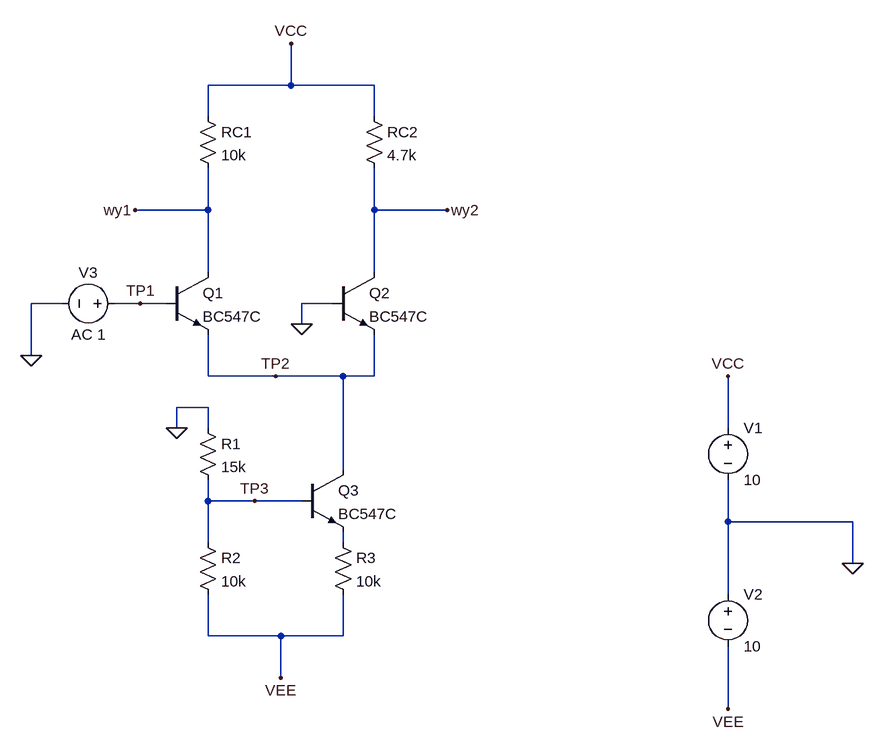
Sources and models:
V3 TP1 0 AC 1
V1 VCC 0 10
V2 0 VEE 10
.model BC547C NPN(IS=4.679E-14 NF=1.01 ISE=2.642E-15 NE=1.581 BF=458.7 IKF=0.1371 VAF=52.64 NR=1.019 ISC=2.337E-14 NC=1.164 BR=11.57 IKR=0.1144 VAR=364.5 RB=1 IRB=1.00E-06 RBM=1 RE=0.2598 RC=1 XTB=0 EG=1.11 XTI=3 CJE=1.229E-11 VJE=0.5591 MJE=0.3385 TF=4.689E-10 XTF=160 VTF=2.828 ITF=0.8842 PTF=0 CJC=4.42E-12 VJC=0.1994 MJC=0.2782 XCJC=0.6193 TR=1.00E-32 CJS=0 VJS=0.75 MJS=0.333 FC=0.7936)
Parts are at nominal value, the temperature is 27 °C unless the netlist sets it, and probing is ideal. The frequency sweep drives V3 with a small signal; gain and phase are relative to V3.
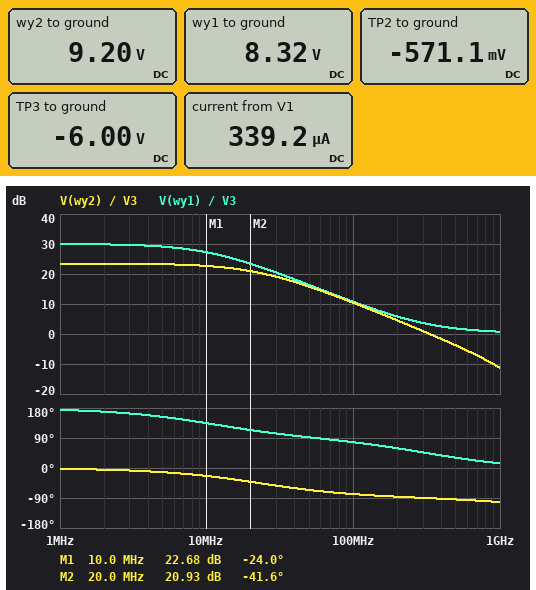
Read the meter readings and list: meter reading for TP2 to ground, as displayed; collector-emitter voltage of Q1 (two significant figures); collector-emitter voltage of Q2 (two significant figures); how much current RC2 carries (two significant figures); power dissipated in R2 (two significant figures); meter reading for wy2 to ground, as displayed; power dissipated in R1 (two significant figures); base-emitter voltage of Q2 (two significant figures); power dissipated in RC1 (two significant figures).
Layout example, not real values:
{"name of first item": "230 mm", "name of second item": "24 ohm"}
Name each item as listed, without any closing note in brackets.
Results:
{"meter reading for TP2 to ground, as displayed": "-571.1 mV", "collector-emitter voltage of Q1": "8.9 V", "collector-emitter voltage of Q2": "9.8 V", "how much current RC2 carries": "170 µA", "power dissipated in R2": "1.6 mW", "meter reading for wy2 to ground, as displayed": "9.20 V", "power dissipated in R1": "2.4 mW", "base-emitter voltage of Q2": "570 mV", "power dissipated in RC1": "280 µW"}
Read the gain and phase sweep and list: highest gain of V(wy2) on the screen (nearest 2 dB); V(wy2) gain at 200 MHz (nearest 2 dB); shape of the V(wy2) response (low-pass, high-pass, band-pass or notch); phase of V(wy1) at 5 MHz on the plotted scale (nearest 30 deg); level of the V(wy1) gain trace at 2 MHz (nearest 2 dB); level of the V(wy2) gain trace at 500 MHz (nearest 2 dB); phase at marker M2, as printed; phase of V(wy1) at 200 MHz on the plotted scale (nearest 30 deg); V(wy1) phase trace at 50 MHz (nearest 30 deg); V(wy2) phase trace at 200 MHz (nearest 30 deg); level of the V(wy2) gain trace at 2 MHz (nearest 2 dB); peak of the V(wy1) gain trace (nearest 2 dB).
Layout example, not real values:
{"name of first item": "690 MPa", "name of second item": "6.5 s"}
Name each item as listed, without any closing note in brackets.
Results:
{"highest gain of V(wy2) on the screen": "24 dB", "V(wy2) gain at 200 MHz": "4 dB", "shape of the V(wy2) response": "low-pass", "phase of V(wy1) at 5 MHz on the plotted scale": "150 deg", "level of the V(wy1) gain trace at 2 MHz": "30 dB", "level of the V(wy2) gain trace at 500 MHz": "-4 dB", "phase at marker M2, as printed": "-41.6 deg", "phase of V(wy1) at 200 MHz on the plotted scale": "60 deg", "V(wy1) phase trace at 50 MHz": "90 deg", "V(wy2) phase trace at 200 MHz": "-90 deg", "level of the V(wy2) gain trace at 2 MHz": "24 dB", "peak of the V(wy1) gain trace": "30 dB"}
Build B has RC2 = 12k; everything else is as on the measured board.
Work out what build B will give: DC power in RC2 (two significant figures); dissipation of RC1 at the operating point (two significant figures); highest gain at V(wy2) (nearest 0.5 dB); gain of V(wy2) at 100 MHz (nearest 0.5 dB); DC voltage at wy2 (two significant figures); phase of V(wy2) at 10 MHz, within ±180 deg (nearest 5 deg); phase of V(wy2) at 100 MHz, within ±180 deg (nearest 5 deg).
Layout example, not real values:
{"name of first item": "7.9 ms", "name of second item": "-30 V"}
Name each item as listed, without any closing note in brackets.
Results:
{"DC power in RC2": "340 µW", "dissipation of RC1 at the operating point": "290 µW", "highest gain at V(wy2)": "31.5 dB", "gain of V(wy2) at 100 MHz": "10.0 dB", "DC voltage at wy2": "8.0 V", "phase of V(wy2) at 10 MHz, within ±180 deg": "-50 deg", "phase of V(wy2) at 100 MHz, within ±180 deg": "-85 deg"}
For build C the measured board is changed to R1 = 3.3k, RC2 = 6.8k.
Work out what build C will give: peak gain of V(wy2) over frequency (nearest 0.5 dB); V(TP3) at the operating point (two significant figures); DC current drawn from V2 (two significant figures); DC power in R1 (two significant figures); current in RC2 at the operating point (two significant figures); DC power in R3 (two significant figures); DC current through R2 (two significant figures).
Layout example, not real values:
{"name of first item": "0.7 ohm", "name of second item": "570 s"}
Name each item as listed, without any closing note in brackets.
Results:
{"peak gain of V(wy2) over frequency": "32.5 dB", "V(TP3) at the operating point": "-2.5 V", "DC current drawn from V2": "1.4 mA", "DC power in R1": "1.9 mW", "current in RC2 at the operating point": "350 µA", "DC power in R3": "4.8 mW", "DC current through R2": "750 µA"}
